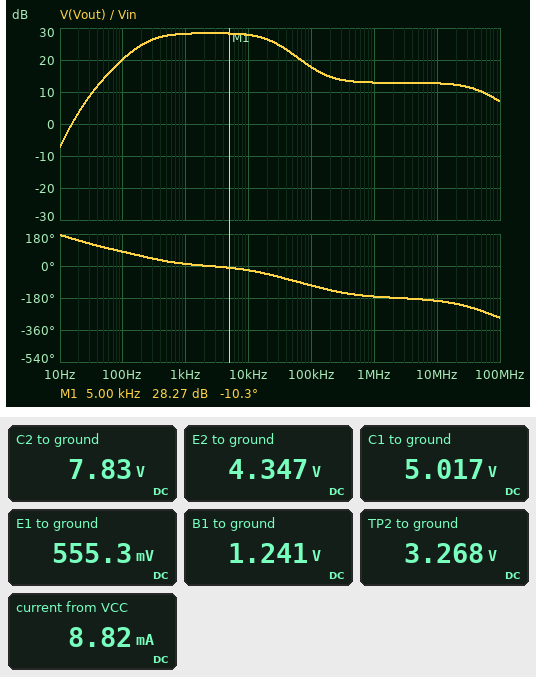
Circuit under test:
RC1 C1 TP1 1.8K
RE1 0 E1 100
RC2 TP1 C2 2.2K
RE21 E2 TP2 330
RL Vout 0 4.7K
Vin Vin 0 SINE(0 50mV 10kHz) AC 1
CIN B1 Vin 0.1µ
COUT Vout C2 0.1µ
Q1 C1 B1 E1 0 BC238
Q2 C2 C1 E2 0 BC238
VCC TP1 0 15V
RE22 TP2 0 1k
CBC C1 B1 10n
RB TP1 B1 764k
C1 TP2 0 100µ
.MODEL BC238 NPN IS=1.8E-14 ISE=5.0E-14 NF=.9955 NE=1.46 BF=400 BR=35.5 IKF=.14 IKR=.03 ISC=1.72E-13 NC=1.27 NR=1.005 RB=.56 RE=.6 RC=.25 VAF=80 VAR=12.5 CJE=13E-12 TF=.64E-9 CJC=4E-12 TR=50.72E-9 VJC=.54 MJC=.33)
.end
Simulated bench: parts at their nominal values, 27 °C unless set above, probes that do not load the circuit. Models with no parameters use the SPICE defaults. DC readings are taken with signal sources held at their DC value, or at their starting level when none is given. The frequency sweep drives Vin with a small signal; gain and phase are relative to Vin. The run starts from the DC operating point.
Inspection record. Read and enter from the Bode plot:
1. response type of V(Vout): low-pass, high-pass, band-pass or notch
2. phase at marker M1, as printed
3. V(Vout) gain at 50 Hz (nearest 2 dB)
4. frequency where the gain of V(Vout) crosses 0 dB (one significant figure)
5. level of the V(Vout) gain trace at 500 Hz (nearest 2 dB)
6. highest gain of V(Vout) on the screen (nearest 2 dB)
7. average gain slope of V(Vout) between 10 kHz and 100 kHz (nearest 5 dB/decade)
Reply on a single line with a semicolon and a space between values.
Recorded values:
band-pass; -10.3 deg; 14 dB; 20 Hz; 28 dB; 28 dB; -10 dB/decade
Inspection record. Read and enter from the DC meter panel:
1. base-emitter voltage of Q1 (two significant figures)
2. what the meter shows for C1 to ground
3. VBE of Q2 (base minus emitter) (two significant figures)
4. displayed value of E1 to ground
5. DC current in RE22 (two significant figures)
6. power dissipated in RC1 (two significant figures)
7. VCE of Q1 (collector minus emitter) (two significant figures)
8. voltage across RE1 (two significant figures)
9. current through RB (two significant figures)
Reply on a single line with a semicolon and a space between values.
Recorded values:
690 mV; 5.017 V; 670 mV; 555.3 mV; 3.3 mA; 55 mW; 4.5 V; 560 mV; 18 µA
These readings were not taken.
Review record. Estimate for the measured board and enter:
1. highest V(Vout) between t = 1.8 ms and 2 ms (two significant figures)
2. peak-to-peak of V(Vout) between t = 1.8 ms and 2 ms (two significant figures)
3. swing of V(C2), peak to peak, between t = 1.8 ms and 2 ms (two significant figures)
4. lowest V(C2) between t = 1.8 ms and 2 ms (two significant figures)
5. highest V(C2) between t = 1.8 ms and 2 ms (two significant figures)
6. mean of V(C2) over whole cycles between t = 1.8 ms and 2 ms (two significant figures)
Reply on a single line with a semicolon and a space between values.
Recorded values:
1.2 V; 2.5 V; 2.5 V; 6.6 V; 9.1 V; 7.8 V
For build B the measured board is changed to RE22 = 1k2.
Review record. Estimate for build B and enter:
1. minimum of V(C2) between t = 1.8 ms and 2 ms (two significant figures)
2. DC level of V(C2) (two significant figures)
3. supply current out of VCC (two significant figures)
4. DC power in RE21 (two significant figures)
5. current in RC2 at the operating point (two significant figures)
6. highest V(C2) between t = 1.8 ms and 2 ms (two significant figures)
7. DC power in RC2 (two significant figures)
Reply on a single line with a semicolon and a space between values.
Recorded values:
7.5 V; 8.8 V; 8.4 mA; 2.7 mW; 2.8 mA; 10 V; 18 mW
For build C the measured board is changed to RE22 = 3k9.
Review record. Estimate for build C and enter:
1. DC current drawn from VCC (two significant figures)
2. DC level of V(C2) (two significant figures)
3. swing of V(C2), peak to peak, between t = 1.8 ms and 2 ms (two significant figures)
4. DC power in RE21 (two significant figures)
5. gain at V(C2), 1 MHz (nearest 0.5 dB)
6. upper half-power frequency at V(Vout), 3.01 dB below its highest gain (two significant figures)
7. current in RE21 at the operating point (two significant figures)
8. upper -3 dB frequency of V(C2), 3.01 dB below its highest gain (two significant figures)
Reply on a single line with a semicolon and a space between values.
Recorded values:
6.6 mA; 13 V; 2.3 V; 360 µW; 12.5 dB; 26 kHz; 1.0 mA; 5.9 kHz
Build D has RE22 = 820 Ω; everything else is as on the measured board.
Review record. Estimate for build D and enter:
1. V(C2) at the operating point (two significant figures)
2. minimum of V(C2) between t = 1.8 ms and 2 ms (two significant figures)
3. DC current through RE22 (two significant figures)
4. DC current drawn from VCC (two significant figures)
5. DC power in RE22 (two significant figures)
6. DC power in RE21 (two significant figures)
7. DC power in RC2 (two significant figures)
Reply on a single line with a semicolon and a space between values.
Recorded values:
6.7 V; 5.5 V; 3.8 mA; 9.3 mA; 12 mW; 4.7 mW; 31 mW
